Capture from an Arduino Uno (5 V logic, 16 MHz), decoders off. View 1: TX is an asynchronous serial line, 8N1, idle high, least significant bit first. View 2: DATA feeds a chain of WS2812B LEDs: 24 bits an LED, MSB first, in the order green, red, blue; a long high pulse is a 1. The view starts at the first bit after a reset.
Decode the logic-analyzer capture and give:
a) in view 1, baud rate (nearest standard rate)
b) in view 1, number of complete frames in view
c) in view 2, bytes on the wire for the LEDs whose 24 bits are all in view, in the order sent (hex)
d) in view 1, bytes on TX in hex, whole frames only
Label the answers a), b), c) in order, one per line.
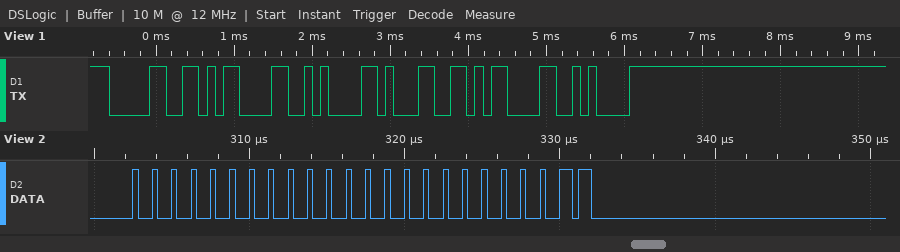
a) 9600 baud
b) 6
c) 00 00 03
d) 30 0D 0A 31 0D 0A
